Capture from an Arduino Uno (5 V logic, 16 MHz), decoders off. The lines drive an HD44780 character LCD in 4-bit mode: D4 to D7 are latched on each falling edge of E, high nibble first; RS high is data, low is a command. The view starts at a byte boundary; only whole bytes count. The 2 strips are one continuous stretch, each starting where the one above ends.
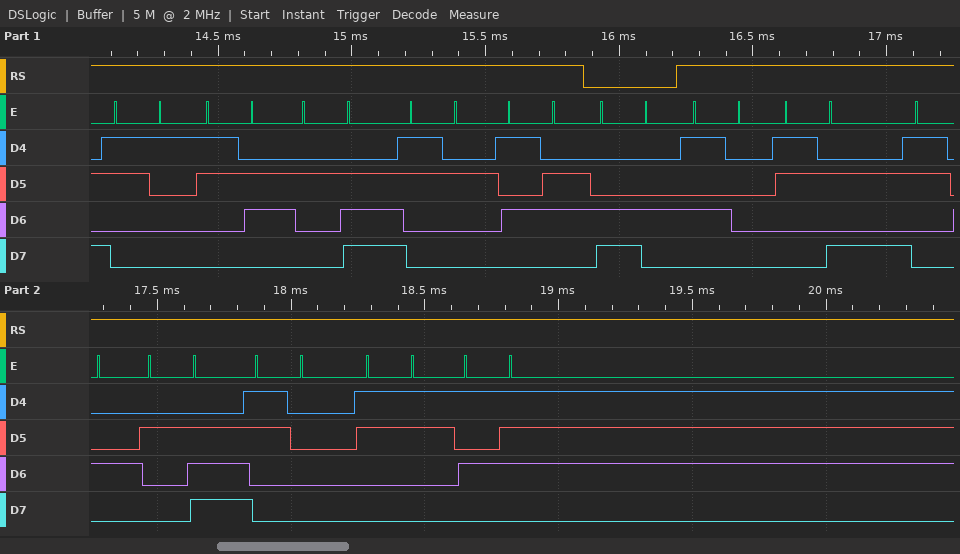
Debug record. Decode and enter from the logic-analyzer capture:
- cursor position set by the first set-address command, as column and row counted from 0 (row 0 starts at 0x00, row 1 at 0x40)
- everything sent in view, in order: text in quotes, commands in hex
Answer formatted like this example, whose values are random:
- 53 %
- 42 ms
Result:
- column 4, row 1
- "16.2V" 0xC4 "P:4.03W"
